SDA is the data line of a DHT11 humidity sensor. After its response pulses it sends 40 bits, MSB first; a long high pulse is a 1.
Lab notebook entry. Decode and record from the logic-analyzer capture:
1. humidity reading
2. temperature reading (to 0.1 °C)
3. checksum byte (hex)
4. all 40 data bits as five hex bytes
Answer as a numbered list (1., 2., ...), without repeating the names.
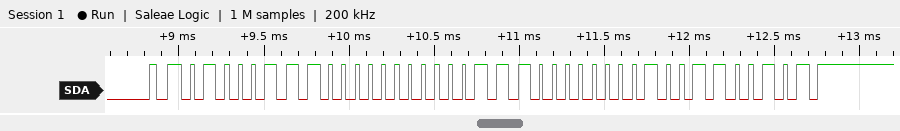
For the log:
1. 71 %
2. 28.2 °C
3. 0x65
4. 47 00 1C 02 65
